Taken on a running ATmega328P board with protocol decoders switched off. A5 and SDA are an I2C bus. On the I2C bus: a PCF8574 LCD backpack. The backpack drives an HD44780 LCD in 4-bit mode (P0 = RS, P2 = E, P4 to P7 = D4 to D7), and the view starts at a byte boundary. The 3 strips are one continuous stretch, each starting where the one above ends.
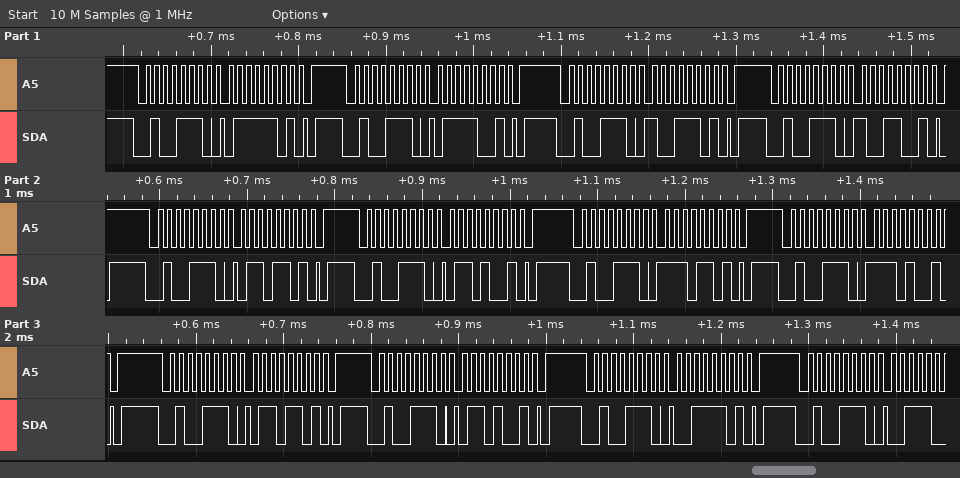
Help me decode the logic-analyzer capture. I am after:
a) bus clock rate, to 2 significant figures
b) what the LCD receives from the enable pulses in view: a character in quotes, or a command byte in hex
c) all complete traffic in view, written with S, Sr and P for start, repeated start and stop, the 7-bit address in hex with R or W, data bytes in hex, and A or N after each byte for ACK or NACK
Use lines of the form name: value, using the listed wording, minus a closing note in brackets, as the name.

bus clock rate, to 2 significant figures: 100 kHz
what the LCD receives from the enable pulses in view: a character in quotes, or a command byte in hex: 'y' 'n'
all complete traffic in view, written with S, Sr and P for start, repeated start and stop, the 7-bit address in hex with R or W, data bytes in hex, and A or N after each byte for ACK or NACK: S 27W A 7D A P S 27W A 79 A P S 27W A 9D A P S 27W A 99 A P S 27W A 6D A P S 27W A 69 A P S 27W A ED A P S 27W A E9 A P S 27W A 6D A P S 27W A 69 A P S 27W A 3D A P S 27W A
